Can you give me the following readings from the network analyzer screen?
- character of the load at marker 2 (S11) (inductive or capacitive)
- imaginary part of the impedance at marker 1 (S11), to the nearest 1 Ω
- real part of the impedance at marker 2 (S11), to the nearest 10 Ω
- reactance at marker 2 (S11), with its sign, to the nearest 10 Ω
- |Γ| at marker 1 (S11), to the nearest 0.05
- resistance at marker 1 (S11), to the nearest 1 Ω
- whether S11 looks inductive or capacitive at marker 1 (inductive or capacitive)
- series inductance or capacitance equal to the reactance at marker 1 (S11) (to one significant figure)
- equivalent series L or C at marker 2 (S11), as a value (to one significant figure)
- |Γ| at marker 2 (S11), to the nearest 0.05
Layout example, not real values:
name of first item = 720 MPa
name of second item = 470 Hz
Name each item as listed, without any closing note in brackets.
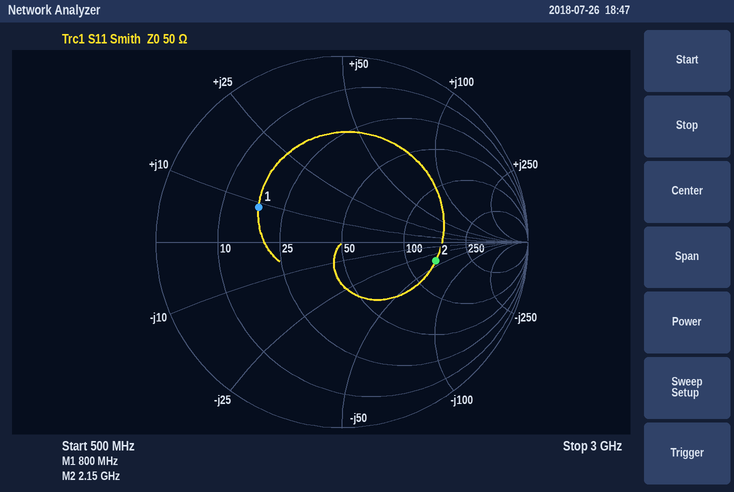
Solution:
character of the load at marker 2 (S11) = capacitive
imaginary part of the impedance at marker 1 (S11), to the nearest 1 Ω = +9 Ω
real part of the impedance at marker 2 (S11), to the nearest 10 Ω = 140 Ω
reactance at marker 2 (S11), with its sign, to the nearest 10 Ω = -40 Ω
|Γ| at marker 1 (S11), to the nearest 0.05 = 0.50
resistance at marker 1 (S11), to the nearest 1 Ω = 18 Ω
whether S11 looks inductive or capacitive at marker 1 = inductive
series inductance or capacitance equal to the reactance at marker 1 (S11) = 2 nH
equivalent series L or C at marker 2 (S11), as a value = 2 pF
|Γ| at marker 2 (S11), to the nearest 0.05 = 0.50
